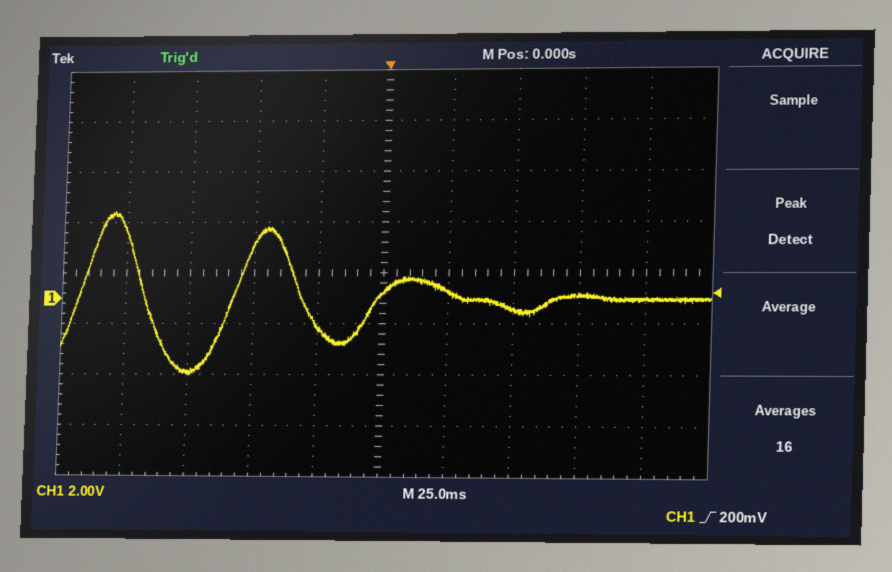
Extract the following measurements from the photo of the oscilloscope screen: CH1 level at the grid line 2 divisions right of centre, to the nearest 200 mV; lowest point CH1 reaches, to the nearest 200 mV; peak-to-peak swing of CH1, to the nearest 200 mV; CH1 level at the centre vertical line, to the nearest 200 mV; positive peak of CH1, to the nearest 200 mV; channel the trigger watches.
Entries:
-400 mV
-3.0 V
6.4 V
200 mV
3.4 V
CH1
